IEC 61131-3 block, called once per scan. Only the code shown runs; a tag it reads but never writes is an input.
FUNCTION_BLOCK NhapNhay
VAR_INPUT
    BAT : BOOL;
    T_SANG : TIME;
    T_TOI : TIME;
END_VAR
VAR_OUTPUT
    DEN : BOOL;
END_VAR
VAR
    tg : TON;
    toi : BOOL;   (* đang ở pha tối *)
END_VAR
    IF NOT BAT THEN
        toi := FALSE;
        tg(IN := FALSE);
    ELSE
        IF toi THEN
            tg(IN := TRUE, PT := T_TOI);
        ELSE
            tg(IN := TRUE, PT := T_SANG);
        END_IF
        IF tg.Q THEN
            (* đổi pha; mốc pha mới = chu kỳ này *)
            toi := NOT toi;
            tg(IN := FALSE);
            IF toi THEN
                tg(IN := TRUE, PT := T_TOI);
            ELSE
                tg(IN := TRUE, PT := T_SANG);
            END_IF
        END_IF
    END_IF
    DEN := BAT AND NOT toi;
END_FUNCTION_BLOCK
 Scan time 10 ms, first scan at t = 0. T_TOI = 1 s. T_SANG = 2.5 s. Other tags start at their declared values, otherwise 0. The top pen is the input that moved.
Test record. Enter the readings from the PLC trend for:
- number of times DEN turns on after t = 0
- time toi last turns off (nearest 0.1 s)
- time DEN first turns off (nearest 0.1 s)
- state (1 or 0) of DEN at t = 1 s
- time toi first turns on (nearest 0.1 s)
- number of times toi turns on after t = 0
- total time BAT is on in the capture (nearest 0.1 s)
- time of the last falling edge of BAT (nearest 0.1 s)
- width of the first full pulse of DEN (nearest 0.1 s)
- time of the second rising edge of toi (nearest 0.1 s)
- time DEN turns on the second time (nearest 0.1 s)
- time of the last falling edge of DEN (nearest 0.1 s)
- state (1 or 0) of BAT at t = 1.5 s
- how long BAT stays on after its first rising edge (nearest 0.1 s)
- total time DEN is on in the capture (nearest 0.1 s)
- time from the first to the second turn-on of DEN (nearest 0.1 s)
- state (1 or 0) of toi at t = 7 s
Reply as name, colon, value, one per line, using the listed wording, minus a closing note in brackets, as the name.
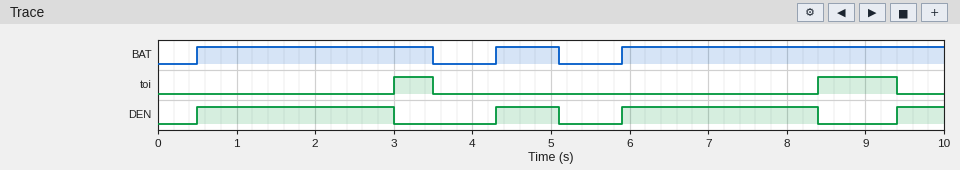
number of times DEN turns on after t = 0: 4
time toi last turns off: 9.4 s
time DEN first turns off: 3.0 s
state (1 or 0) of DEN at t = 1 s: 1
time toi first turns on: 3.0 s
number of times toi turns on after t = 0: 2
total time BAT is on in the capture: 7.9 s
time of the last falling edge of BAT: 5.1 s
width of the first full pulse of DEN: 2.5 s
time of the second rising edge of toi: 8.4 s
time DEN turns on the second time: 4.3 s
time of the last falling edge of DEN: 8.4 s
state (1 or 0) of BAT at t = 1.5 s: 1
how long BAT stays on after its first rising edge: 3.0 s
total time DEN is on in the capture: 6.4 s
time from the first to the second turn-on of DEN: 3.8 s
state (1 or 0) of toi at t = 7 s: 0
